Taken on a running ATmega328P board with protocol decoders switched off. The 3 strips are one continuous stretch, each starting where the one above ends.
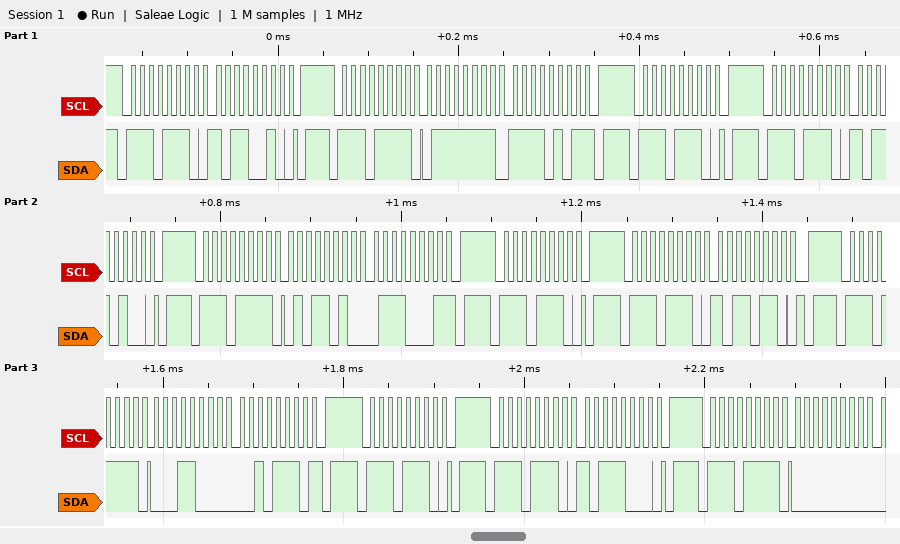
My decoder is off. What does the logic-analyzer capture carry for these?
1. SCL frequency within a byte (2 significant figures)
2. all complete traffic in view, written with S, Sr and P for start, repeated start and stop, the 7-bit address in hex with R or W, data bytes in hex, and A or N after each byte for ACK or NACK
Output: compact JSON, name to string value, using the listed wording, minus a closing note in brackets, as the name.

{"SCL frequency within a byte": "100 kHz", "all complete traffic in view, written with S, Sr and P for start, repeated start and stop, the 7-bit address in hex with R or W, data bytes in hex, and A or N after each byte for ACK or NACK": "S 77W A B2 A P S 77R A 7F A F5 N P S 77W A P S 77W A B4 A P S 77R A 5A A 71 N P S 77W A P S 77W A B6 A P S 77R A 18 A 2E N P S 77W A P S 77W A B8 A P S 77R A 00 A"}
